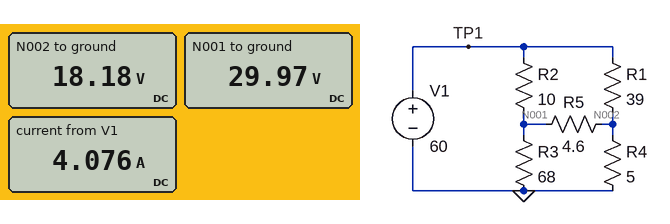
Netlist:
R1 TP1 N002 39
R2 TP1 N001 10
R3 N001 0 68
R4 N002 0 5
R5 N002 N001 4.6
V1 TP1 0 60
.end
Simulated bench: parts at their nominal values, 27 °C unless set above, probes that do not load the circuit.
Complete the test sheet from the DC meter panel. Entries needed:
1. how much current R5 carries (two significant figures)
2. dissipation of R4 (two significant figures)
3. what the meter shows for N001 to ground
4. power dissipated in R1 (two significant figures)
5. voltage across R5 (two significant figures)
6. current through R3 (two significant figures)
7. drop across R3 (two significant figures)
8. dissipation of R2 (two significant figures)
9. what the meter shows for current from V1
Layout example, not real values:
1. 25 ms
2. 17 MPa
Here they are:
1. 2.6 A
2. 66 W
3. 29.97 V
4. 45 W
5. 12 V
6. 440 mA
7. 30 V
8. 90 W
9. 4.076 A
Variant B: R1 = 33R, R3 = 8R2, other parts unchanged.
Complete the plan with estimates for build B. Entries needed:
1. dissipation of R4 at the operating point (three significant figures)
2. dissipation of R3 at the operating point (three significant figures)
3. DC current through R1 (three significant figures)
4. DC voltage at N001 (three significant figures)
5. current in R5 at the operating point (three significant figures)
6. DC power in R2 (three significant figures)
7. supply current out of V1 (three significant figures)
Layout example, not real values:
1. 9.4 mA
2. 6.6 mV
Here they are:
1. 39.6 W
2. 51.9 W
3. 1.39 A
4. 20.6 V
5. 1.42 A
6. 155 W
7. 5.33 A
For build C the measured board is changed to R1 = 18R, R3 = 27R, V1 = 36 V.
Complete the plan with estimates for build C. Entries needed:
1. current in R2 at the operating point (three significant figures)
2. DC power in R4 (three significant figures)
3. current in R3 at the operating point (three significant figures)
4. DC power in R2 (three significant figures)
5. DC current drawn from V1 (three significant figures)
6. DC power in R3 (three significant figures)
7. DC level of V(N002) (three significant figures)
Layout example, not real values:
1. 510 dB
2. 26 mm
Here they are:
1. 1.82 A
2. 30.7 W
3. 658 mA
4. 33.3 W
5. 3.14 A
6. 11.7 W
7. 12.4 V
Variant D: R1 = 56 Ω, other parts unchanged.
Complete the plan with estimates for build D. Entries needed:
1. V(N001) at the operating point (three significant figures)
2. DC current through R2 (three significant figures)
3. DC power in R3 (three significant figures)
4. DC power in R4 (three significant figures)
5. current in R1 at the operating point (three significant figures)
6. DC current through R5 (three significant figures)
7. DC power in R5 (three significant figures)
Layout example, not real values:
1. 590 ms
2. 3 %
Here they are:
1. 29.2 V
2. 3.08 A
3. 12.6 W
4. 58.2 W
5. 767 mA
6. 2.65 A
7. 32.2 W
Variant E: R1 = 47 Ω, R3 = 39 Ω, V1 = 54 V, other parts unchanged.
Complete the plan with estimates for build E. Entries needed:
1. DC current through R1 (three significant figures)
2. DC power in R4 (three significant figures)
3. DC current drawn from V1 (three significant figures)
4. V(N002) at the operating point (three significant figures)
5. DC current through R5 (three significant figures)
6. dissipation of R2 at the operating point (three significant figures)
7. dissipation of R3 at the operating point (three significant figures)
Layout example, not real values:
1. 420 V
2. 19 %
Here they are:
1. 826 mA
2. 46.2 W
3. 3.69 A
4. 15.2 V
5. 2.21 A
6. 82.0 W
7. 16.5 W
